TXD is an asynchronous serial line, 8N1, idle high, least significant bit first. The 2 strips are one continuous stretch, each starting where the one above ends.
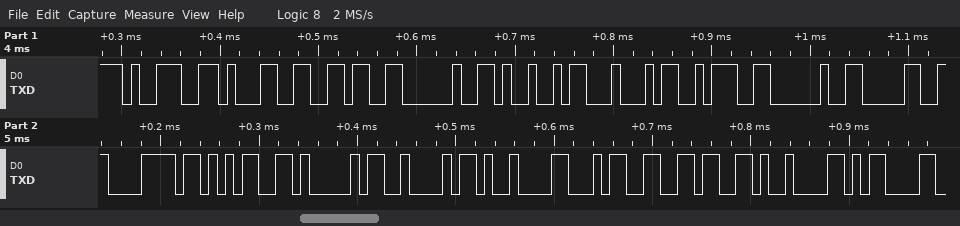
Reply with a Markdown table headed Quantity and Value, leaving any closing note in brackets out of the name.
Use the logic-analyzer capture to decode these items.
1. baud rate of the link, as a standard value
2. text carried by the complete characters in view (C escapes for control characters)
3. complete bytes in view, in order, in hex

| Quantity | Value |
|---|---|
| baud rate of the link, as a standard value | 115200 baud |
| text carried by the complete characters in view | "916 ID: 0x5AB\t46\t\r" |
| complete bytes in view, in order, in hex | 39 31 36 20 49 44 3A 20 30 78 35 41 42 09 34 36 09 0D |
